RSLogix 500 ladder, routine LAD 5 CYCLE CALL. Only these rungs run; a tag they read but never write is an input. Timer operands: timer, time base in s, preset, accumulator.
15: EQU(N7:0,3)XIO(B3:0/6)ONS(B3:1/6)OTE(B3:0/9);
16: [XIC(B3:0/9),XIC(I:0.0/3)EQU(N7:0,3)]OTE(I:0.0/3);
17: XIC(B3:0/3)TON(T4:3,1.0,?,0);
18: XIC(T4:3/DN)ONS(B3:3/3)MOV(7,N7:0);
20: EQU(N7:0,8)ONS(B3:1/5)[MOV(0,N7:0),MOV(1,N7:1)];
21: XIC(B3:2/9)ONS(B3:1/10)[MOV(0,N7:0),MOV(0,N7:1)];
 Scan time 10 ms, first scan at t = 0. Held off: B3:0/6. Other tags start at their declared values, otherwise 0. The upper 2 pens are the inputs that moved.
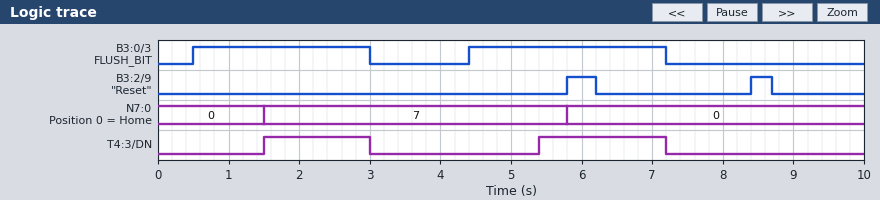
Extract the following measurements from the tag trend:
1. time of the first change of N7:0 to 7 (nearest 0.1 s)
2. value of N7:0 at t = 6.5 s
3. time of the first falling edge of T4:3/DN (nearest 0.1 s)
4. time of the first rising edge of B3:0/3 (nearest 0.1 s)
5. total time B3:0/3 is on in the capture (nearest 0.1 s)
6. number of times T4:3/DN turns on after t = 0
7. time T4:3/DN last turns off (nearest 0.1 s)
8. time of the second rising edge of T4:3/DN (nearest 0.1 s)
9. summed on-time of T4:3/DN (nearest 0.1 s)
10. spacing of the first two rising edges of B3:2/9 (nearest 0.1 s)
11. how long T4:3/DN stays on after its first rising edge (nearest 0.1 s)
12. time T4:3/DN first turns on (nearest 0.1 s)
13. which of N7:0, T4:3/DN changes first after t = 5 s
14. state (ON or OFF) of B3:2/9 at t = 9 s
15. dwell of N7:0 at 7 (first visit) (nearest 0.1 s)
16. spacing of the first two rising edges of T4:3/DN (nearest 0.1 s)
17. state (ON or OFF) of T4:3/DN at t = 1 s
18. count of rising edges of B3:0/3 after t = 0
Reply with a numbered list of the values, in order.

1. 1.5 s
2. 0
3. 3.0 s
4. 0.5 s
5. 5.3 s
6. 2
7. 7.2 s
8. 5.4 s
9. 3.3 s
10. 2.6 s
11. 1.5 s
12. 1.5 s
13. T4:3/DN
14. OFF
15. 4.3 s
16. 3.9 s
17. OFF
18. 2
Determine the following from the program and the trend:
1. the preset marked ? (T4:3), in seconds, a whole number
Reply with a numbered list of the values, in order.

1. 1 s
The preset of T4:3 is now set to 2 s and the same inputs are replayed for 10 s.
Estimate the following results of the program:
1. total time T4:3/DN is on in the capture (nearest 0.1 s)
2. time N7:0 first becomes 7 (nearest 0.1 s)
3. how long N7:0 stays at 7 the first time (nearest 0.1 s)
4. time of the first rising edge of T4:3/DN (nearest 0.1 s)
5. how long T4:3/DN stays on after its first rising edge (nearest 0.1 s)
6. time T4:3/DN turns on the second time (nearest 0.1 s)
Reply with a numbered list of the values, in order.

1. 1.3 s
2. 2.5 s
3. 3.3 s
4. 2.5 s
5. 0.5 s
6. 6.4 s
